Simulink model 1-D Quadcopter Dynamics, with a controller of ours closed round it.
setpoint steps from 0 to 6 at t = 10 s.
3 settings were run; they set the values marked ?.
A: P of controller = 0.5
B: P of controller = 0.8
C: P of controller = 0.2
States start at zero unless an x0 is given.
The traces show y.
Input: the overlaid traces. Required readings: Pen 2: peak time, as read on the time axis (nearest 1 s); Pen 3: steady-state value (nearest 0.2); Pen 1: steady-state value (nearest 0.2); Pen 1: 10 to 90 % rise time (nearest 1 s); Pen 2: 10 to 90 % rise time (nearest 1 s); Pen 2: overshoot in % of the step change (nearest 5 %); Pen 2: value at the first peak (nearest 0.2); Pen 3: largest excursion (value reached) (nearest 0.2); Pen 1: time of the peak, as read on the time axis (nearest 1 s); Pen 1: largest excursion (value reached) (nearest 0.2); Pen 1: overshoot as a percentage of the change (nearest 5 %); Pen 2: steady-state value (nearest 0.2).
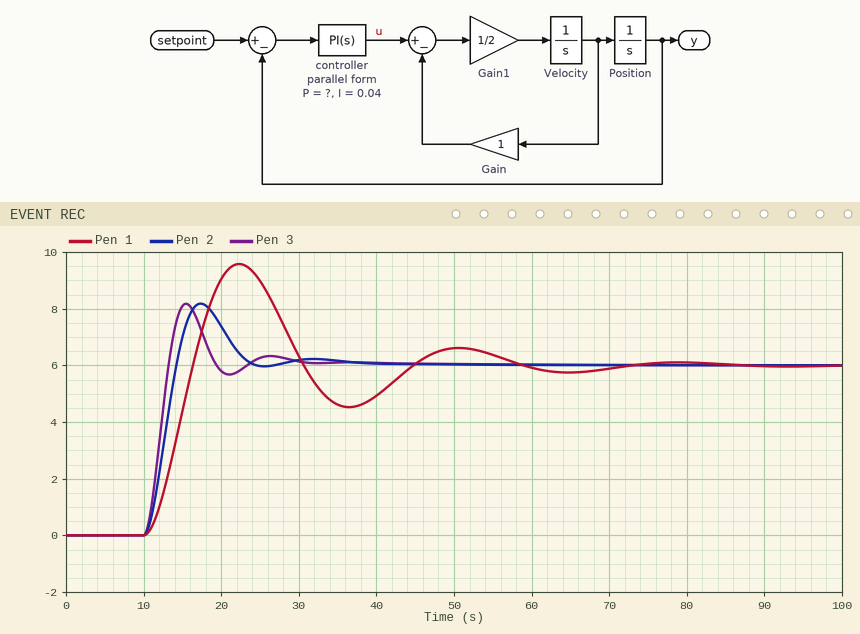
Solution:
17 s
6.0
6.0
4 s
3 s
35 %
8.2
8.2
22 s
9.6
60 %
6.0
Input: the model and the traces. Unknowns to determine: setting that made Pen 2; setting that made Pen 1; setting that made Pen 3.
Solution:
A
C
B
